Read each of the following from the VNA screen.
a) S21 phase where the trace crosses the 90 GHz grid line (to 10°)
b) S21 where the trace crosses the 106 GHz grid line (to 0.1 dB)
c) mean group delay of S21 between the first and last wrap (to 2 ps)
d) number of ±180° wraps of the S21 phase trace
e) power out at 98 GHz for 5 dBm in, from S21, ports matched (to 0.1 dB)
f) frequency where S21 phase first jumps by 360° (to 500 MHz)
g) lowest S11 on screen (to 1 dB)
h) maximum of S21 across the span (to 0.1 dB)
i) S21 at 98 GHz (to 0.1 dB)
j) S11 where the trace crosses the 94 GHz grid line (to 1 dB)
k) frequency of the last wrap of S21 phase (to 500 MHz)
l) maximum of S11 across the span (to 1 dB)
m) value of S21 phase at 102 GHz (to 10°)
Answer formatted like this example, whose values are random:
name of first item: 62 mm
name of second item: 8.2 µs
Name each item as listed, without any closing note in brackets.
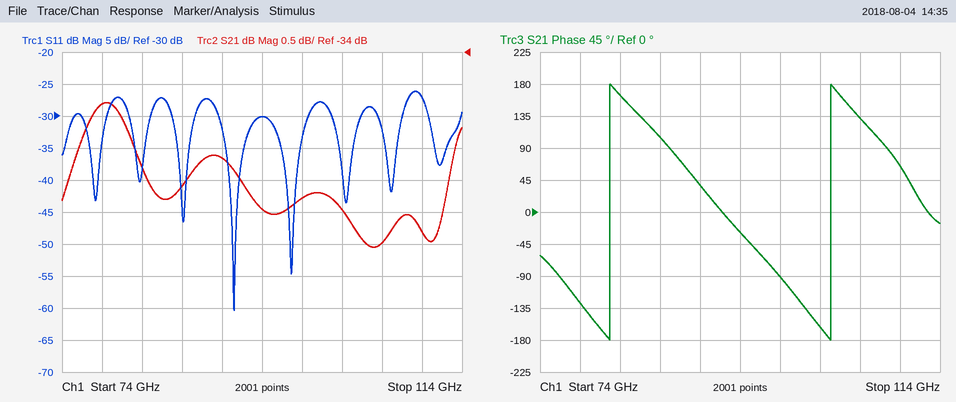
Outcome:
S21 phase where the trace crosses the 90 GHz grid line: 40°
S21 where the trace crosses the 106 GHz grid line: -37.0 dB
mean group delay of S21 between the first and last wrap: 46 ps
number of ±180° wraps of the S21 phase trace: 2
power out at 98 GHz for 5 dBm in, from S21, ports matched: -31.3 dBm
frequency where S21 phase first jumps by 360°: 81.0 GHz
lowest S11 on screen: -60 dB
maximum of S21 across the span: -34.8 dB
S21 at 98 GHz: -36.3 dB
S11 where the trace crosses the 94 GHz grid line: -30 dB
frequency of the last wrap of S21 phase: 103.0 GHz
maximum of S11 across the span: -26 dB
value of S21 phase at 102 GHz: -160°
